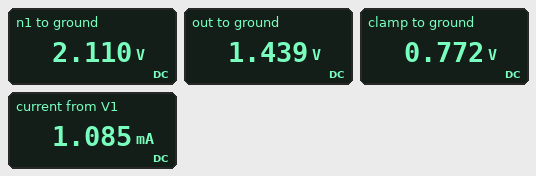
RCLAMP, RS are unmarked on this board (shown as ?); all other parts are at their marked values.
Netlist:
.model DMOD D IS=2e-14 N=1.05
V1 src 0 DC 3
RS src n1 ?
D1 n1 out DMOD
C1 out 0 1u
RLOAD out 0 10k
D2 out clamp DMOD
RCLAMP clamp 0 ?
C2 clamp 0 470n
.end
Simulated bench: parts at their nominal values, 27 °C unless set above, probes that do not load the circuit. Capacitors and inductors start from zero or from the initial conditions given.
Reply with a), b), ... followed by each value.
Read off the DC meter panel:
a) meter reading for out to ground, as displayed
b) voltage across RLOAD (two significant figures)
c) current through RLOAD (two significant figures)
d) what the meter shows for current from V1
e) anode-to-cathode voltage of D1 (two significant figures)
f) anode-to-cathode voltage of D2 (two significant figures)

a) 1.439 V
b) 1.4 V
c) 140 µA
d) 1.085 mA
e) 670 mV
f) 670 mV
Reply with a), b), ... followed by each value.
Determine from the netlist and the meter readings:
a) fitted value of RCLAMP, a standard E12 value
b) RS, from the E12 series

a) 820 Ω
b) 820 Ω
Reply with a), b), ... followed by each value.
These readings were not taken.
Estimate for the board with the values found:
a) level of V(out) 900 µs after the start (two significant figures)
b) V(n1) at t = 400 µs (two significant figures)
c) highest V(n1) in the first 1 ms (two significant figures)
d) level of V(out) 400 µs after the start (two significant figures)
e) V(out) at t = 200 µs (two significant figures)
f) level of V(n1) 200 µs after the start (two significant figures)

a) 1.2 V
b) 1.5 V
c) 1.9 V
d) 800 mV
e) 490 mV
f) 1.2 V
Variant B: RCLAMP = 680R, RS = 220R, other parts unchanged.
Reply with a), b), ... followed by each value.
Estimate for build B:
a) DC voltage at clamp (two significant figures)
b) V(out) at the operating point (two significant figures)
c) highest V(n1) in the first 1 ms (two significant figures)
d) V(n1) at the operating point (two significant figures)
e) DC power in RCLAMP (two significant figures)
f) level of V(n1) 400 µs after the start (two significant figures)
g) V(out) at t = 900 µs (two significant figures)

a) 1.2 V
b) 1.9 V
c) 2.5 V
d) 2.6 V
e) 2.1 mW
f) 2.3 V
g) 1.8 V
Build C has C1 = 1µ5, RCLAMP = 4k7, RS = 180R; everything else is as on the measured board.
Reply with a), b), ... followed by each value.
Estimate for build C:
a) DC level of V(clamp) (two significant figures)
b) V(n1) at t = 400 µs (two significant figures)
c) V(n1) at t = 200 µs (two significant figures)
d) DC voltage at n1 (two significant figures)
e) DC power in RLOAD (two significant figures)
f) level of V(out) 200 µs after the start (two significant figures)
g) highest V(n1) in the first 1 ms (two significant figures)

a) 1.6 V
b) 2.3 V
c) 1.8 V
d) 2.9 V
e) 500 µW
f) 1.1 V
g) 2.8 V
